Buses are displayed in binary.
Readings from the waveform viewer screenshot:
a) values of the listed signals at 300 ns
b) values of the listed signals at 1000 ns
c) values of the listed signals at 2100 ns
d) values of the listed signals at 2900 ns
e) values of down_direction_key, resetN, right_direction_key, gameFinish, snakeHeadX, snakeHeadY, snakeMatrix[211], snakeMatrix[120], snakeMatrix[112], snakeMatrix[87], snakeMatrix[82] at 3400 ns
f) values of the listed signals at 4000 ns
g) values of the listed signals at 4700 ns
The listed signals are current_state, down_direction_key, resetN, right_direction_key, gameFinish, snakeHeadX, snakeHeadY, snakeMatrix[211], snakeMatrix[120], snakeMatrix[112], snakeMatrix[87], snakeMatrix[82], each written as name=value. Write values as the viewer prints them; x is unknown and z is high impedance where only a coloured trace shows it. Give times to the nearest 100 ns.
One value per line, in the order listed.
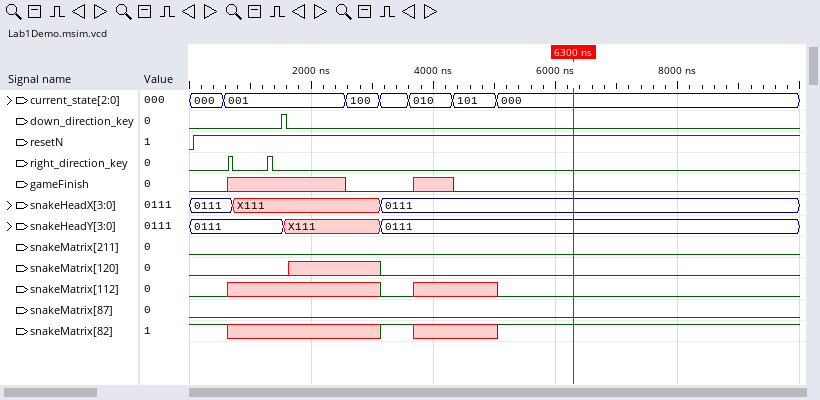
current_state=000, down_direction_key=0, resetN=1, right_direction_key=0, gameFinish=0, snakeHeadX=0111, snakeHeadY=0111, snakeMatrix[211]=0, snakeMatrix[120]=0, snakeMatrix[112]=0, snakeMatrix[87]=0, snakeMatrix[82]=1
current_state=001, down_direction_key=0, resetN=1, right_direction_key=0, gameFinish=x, snakeHeadX=X111, snakeHeadY=0111, snakeMatrix[211]=0, snakeMatrix[120]=0, snakeMatrix[112]=x, snakeMatrix[87]=0, snakeMatrix[82]=x
current_state=001, down_direction_key=0, resetN=1, right_direction_key=0, gameFinish=x, snakeHeadX=X111, snakeHeadY=X111, snakeMatrix[211]=0, snakeMatrix[120]=x, snakeMatrix[112]=x, snakeMatrix[87]=0, snakeMatrix[82]=x
current_state=100, down_direction_key=0, resetN=1, right_direction_key=0, gameFinish=0, snakeHeadX=X111, snakeHeadY=X111, snakeMatrix[211]=0, snakeMatrix[120]=x, snakeMatrix[112]=x, snakeMatrix[87]=0, snakeMatrix[82]=x
down_direction_key=0, resetN=1, right_direction_key=0, gameFinish=0, snakeHeadX=0111, snakeHeadY=0111, snakeMatrix[211]=0, snakeMatrix[120]=0, snakeMatrix[112]=0, snakeMatrix[87]=0, snakeMatrix[82]=1
current_state=010, down_direction_key=0, resetN=1, right_direction_key=0, gameFinish=x, snakeHeadX=0111, snakeHeadY=0111, snakeMatrix[211]=0, snakeMatrix[120]=0, snakeMatrix[112]=x, snakeMatrix[87]=0, snakeMatrix[82]=x
current_state=101, down_direction_key=0, resetN=1, right_direction_key=0, gameFinish=0, snakeHeadX=0111, snakeHeadY=0111, snakeMatrix[211]=0, snakeMatrix[120]=0, snakeMatrix[112]=x, snakeMatrix[87]=0, snakeMatrix[82]=x
